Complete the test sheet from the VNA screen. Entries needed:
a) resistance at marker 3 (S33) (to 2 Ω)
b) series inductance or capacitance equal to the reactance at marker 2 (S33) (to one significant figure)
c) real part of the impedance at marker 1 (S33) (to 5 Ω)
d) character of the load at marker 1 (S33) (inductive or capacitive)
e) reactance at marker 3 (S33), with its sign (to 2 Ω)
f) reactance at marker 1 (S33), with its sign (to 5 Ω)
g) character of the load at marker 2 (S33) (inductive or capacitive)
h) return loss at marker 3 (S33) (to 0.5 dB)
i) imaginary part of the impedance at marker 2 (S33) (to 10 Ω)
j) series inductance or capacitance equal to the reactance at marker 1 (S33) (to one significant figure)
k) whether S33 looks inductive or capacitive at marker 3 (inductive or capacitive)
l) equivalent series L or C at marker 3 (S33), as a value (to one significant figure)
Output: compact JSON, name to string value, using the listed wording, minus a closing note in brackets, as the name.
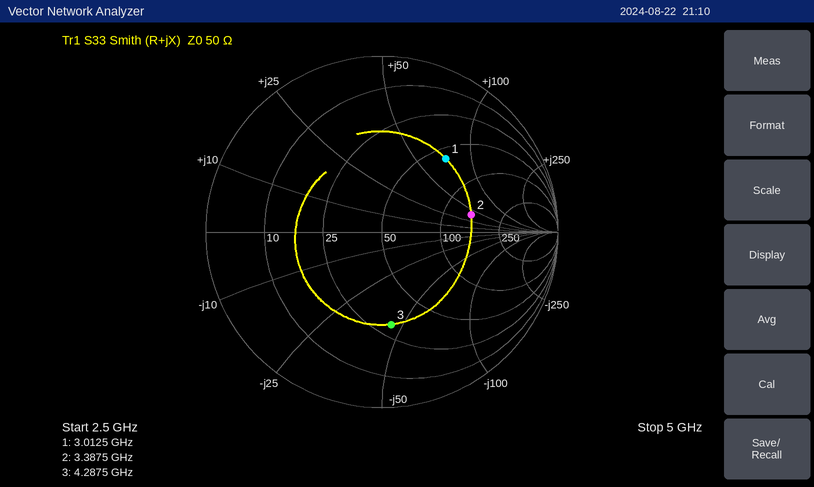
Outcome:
{"resistance at marker 3 (S33)": "30 Ω", "series inductance or capacitance equal to the reactance at marker 2 (S33)": "2 nH", "real part of the impedance at marker 1 (S33)": "60 Ω", "character of the load at marker 1 (S33)": "inductive", "reactance at marker 3 (S33), with its sign": "-44 Ω", "reactance at marker 1 (S33), with its sign": "+70 Ω", "character of the load at marker 2 (S33)": "inductive", "return loss at marker 3 (S33)": "5.5 dB", "imaginary part of the impedance at marker 2 (S33)": "+40 Ω", "series inductance or capacitance equal to the reactance at marker 1 (S33)": "4 nH", "whether S33 looks inductive or capacitive at marker 3": "capacitive", "equivalent series L or C at marker 3 (S33), as a value": "800 fF"}
